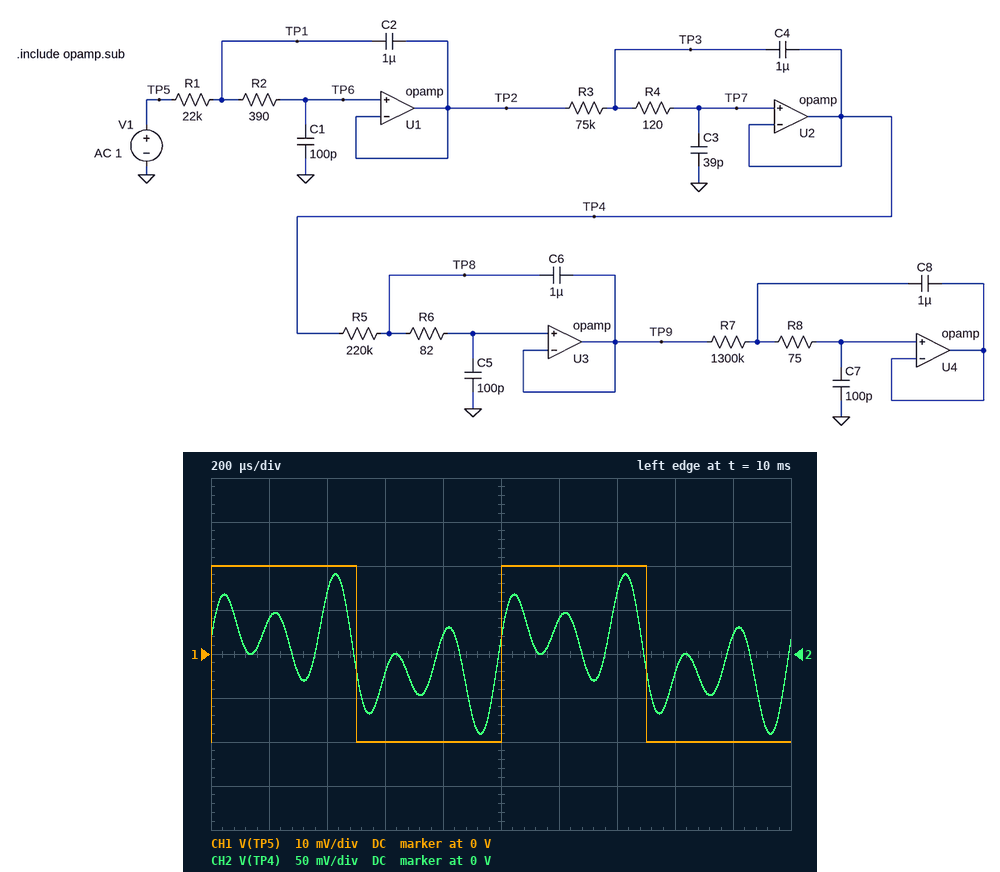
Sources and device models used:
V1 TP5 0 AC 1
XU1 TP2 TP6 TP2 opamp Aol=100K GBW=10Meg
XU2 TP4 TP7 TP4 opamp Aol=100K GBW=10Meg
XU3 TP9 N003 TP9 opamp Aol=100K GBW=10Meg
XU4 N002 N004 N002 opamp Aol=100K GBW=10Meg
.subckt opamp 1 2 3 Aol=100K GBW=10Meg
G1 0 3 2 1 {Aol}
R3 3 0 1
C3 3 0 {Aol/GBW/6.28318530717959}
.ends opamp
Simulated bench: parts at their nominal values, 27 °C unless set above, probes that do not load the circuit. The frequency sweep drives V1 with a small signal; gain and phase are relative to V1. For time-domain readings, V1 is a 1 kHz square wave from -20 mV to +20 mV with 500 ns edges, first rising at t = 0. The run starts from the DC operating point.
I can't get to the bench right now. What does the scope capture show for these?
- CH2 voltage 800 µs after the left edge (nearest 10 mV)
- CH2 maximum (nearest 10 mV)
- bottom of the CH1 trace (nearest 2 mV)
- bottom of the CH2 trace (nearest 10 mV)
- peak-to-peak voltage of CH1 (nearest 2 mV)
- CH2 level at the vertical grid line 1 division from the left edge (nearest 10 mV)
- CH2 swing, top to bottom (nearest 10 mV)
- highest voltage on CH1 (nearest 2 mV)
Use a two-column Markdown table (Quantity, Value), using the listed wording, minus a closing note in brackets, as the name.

| Quantity | Value |
|---|---|
| CH2 voltage 800 µs after the left edge | 20 mV |
| CH2 maximum | 90 mV |
| bottom of the CH1 trace | -20 mV |
| bottom of the CH2 trace | -90 mV |
| peak-to-peak voltage of CH1 | 40 mV |
| CH2 level at the vertical grid line 1 division from the left edge | 40 mV |
| CH2 swing, top to bottom | 180 mV |
| highest voltage on CH1 | 20 mV |
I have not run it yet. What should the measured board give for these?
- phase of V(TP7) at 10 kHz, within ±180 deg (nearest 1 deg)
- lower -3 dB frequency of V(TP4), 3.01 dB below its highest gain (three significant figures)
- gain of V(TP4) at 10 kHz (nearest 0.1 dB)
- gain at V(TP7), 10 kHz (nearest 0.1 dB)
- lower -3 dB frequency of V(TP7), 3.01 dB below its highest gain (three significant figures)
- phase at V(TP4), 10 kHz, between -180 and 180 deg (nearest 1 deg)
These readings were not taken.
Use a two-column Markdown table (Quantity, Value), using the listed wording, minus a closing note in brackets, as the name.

| Quantity | Value |
|---|---|
| phase of V(TP7) at 10 kHz, within ±180 deg | 5 deg |
| lower -3 dB frequency of V(TP4), 3.01 dB below its highest gain | 3.94 kHz |
| gain of V(TP4) at 10 kHz | -25.7 dB |
| gain at V(TP7), 10 kHz | -25.7 dB |
| lower -3 dB frequency of V(TP7), 3.01 dB below its highest gain | 3.94 kHz |
| phase at V(TP4), 10 kHz, between -180 and 180 deg | 5 deg |
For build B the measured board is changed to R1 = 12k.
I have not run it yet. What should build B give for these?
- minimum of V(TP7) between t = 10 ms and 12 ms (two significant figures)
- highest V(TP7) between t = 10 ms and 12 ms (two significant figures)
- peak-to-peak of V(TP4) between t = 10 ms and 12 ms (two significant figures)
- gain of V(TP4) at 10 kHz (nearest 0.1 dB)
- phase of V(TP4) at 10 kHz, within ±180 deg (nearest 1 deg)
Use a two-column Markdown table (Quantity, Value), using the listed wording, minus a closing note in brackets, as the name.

| Quantity | Value |
|---|---|
| minimum of V(TP7) between t = 10 ms and 12 ms | -65 mV |
| highest V(TP7) between t = 10 ms and 12 ms | 65 mV |
| peak-to-peak of V(TP4) between t = 10 ms and 12 ms | 130 mV |
| gain of V(TP4) at 10 kHz | -18.3 dB |
| phase of V(TP4) at 10 kHz, within ±180 deg | 6 deg |
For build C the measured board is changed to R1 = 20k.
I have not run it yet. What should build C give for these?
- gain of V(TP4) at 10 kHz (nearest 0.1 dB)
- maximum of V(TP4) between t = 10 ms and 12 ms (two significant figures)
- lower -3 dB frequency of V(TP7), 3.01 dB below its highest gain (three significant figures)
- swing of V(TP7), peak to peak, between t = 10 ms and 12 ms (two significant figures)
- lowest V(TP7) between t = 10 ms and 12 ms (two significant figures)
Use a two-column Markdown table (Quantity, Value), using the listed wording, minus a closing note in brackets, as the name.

| Quantity | Value |
|---|---|
| gain of V(TP4) at 10 kHz | -24.6 dB |
| maximum of V(TP4) between t = 10 ms and 12 ms | 130 mV |
| lower -3 dB frequency of V(TP7), 3.01 dB below its highest gain | 3.91 kHz |
| swing of V(TP7), peak to peak, between t = 10 ms and 12 ms | 260 mV |
| lowest V(TP7) between t = 10 ms and 12 ms | -130 mV |
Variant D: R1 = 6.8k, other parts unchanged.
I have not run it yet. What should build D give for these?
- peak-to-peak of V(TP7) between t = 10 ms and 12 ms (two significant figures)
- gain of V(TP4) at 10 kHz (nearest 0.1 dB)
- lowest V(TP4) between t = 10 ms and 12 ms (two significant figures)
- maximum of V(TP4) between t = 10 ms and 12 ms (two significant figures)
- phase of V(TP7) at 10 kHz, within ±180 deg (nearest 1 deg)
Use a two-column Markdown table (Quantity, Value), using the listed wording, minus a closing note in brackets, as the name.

| Quantity | Value |
|---|---|
| peak-to-peak of V(TP7) between t = 10 ms and 12 ms | 110 mV |
| gain of V(TP4) at 10 kHz | -7.7 dB |
| lowest V(TP4) between t = 10 ms and 12 ms | -57 mV |
| maximum of V(TP4) between t = 10 ms and 12 ms | 57 mV |
| phase of V(TP7) at 10 kHz, within ±180 deg | 9 deg |
